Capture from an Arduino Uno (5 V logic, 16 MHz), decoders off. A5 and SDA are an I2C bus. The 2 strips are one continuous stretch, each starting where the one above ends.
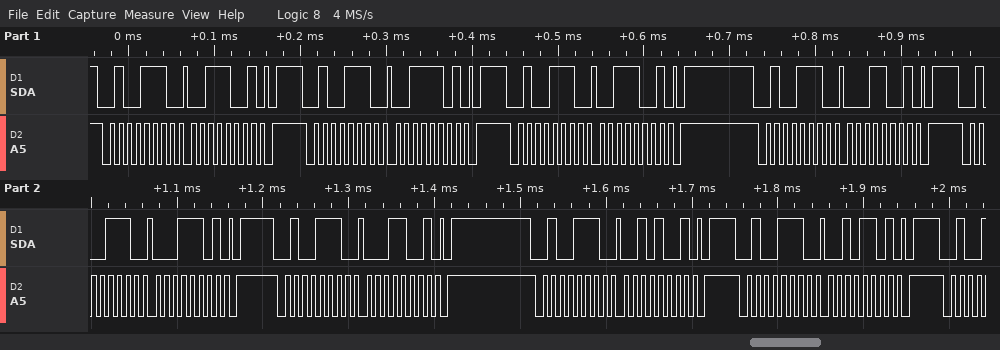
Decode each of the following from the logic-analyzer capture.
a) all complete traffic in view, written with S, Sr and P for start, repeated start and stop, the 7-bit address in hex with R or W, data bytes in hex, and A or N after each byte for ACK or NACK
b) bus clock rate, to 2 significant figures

S 27W A 39 A P S 27W A 3D A P S 27W A 39 A P S 27W A 19 A P S 27W A 1D A P S 27W A 19 A P S 27W A 29 A P S 27W A 2D A P
100 kHz
